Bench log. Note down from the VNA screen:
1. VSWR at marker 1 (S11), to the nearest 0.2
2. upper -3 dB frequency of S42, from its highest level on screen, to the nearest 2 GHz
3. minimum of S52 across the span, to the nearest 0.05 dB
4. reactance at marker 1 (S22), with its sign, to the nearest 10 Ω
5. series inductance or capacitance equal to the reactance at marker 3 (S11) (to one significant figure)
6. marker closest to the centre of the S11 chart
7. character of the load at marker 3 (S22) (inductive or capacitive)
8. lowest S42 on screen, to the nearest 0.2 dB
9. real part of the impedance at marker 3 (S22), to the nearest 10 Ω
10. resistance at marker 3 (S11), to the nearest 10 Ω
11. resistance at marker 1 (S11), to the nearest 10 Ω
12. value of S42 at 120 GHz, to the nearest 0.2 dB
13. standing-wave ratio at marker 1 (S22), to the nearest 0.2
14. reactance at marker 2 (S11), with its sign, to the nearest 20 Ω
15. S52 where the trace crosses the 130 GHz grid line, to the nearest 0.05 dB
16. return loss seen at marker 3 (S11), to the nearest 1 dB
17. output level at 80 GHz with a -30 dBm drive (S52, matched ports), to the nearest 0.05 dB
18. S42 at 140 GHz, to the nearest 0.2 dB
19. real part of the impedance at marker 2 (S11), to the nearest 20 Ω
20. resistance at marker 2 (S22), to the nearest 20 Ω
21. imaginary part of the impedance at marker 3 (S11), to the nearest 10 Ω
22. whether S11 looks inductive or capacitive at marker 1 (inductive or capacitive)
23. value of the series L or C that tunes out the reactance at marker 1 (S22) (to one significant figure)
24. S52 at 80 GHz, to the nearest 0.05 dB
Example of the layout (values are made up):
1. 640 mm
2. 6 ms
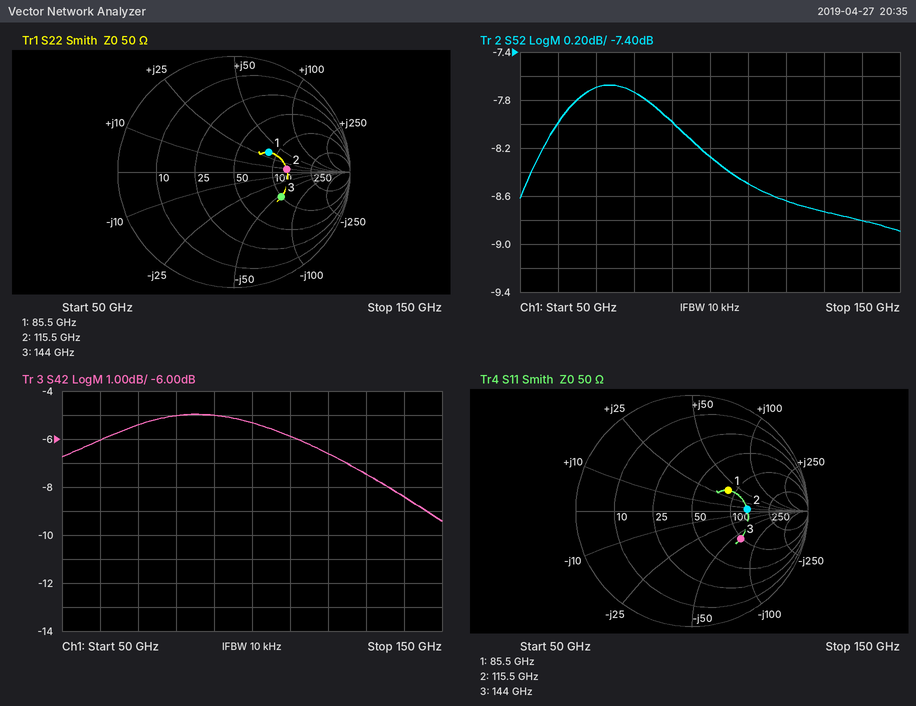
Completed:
1. 2.2
2. 136 GHz
3. -8.90 dB
4. +30 Ω
5. 20 fF
6. marker 1
7. capacitive
8. -9.4 dB
9. 100 Ω
10. 100 Ω
11. 90 Ω
12. -6.6 dB
13. 2.0
14. 0 Ω
15. -8.75 dB
16. 6 dB
17. -37.75 dBm
18. -8.4 dB
19. 140 Ω
20. 140 Ω
21. -60 Ω
22. inductive
23. 60 fF
24. -7.75 dB
